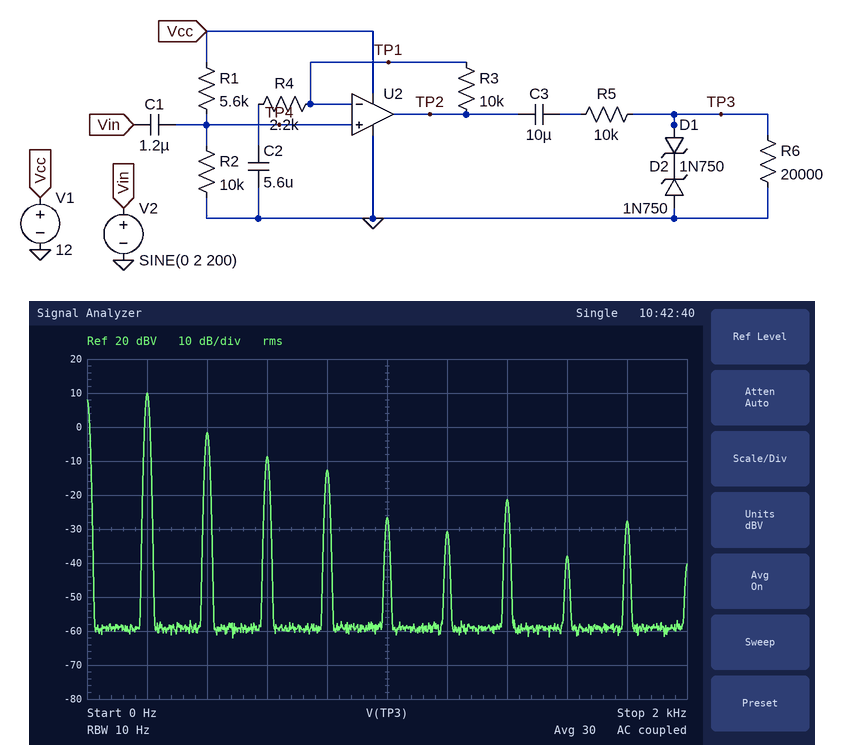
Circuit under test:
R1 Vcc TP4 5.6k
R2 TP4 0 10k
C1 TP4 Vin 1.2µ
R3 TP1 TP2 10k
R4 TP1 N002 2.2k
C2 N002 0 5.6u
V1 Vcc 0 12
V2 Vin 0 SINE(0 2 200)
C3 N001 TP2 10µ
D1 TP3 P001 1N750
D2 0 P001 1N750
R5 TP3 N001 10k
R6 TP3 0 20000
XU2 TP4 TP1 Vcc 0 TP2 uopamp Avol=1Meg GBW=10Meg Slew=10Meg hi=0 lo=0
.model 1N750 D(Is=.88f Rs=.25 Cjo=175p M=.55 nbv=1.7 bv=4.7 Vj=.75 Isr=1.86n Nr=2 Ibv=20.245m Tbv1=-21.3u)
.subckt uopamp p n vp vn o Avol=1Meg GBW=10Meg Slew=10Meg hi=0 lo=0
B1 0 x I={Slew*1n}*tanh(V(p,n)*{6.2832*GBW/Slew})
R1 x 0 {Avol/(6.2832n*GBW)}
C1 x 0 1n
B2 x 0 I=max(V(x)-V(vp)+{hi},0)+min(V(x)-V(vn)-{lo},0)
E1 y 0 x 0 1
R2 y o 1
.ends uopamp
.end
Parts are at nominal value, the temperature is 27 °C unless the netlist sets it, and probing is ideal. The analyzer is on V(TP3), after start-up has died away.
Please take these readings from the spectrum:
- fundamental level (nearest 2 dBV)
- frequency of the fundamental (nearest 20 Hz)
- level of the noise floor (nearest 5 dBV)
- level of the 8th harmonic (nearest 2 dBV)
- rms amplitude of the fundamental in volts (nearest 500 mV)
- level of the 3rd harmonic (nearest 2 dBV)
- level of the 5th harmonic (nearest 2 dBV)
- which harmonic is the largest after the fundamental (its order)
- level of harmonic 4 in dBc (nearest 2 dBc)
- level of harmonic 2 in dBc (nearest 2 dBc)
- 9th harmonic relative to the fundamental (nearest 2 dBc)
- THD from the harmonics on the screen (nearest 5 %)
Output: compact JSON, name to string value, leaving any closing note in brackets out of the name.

{"fundamental level": "10 dBV", "frequency of the fundamental": "200 Hz", "level of the noise floor": "-60 dBV", "level of the 8th harmonic": "-38 dBV", "rms amplitude of the fundamental in volts": "3.0 V", "level of the 3rd harmonic": "-8 dBV", "level of the 5th harmonic": "-26 dBV", "which harmonic is the largest after the fundamental": "2", "level of harmonic 4 in dBc": "-22 dBc", "level of harmonic 2 in dBc": "-12 dBc", "9th harmonic relative to the fundamental": "-38 dBc", "THD from the harmonics on the screen": "30 %"}
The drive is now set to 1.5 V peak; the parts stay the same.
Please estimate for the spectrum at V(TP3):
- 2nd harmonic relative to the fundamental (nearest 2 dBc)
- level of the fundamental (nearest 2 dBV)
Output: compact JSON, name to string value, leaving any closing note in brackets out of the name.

{"2nd harmonic relative to the fundamental": "-14 dBc", "level of the fundamental": "10 dBV"}
